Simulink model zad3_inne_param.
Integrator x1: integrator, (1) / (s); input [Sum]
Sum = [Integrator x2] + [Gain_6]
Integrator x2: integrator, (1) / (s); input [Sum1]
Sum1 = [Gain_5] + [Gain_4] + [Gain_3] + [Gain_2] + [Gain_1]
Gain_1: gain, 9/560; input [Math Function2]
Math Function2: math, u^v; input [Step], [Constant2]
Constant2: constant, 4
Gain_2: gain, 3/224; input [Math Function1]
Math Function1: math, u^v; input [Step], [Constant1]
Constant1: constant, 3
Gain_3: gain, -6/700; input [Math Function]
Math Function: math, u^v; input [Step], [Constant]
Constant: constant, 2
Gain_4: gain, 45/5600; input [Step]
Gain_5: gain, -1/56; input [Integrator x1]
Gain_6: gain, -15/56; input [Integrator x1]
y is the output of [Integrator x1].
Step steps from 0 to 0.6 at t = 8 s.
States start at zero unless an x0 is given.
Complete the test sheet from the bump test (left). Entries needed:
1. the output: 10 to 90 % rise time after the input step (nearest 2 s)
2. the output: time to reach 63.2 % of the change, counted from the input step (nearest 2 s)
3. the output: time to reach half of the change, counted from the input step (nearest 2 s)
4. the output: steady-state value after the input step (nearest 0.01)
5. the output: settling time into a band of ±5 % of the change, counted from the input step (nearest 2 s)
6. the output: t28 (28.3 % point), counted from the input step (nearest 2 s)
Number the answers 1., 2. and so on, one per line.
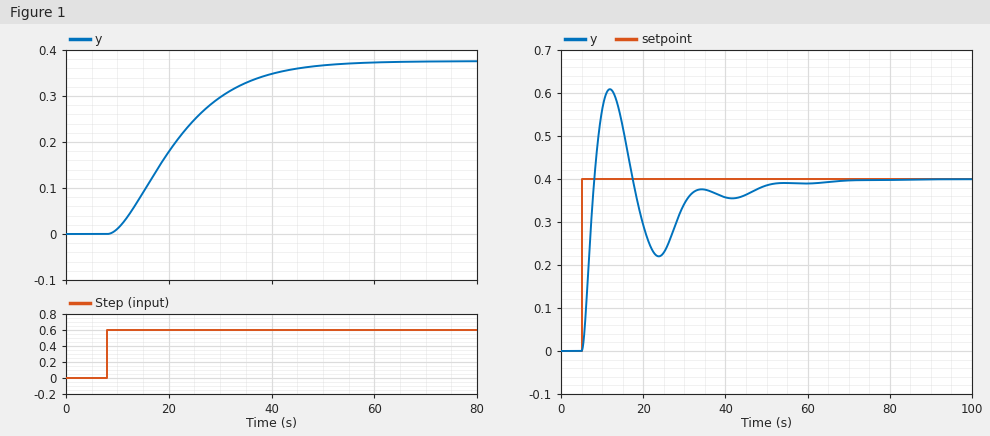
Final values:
1. 26 s
2. 16 s
3. 12 s
4. 0.38
5. 36 s
6. 8 s
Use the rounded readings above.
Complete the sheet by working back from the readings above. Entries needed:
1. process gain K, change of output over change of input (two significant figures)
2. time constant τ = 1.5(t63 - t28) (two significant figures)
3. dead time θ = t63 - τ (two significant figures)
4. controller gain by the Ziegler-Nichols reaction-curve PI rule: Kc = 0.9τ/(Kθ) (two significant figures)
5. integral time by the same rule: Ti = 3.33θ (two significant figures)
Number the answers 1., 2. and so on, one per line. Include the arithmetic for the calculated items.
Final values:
1. (0.38 - 0) / 0.6 = 0.63
2. 1.5 × (16 - 8) = 12 s
3. 16 - 12 = 4.0 s
4. 0.9 × 12 / (0.63 × 4) = 4.3
5. 3.33 × 4 = 13 s
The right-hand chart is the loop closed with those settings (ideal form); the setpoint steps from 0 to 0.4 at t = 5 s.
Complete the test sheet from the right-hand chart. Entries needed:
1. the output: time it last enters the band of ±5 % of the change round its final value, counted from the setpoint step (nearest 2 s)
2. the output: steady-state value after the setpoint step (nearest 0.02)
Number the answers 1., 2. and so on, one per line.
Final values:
1. 44 s
2. 0.40
